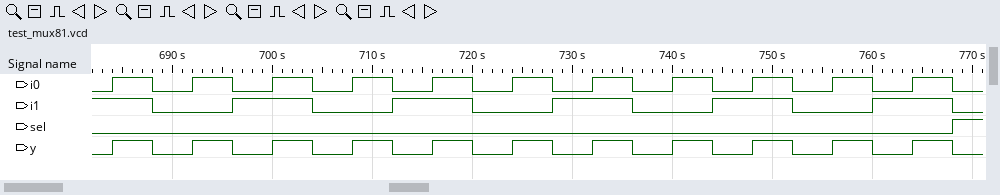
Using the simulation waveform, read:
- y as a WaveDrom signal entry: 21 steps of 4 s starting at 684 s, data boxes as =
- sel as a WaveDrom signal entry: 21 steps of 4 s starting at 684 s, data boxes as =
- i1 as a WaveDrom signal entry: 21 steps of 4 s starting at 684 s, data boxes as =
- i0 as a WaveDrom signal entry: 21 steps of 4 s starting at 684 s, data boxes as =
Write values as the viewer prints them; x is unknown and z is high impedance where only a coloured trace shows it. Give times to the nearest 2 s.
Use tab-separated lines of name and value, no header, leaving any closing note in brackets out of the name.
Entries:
y as a WaveDrom signal entry: 21 steps of 4 s starting at 684 s, data boxes as =	{name: 'y', wave: '101010101010101010101'}
sel as a WaveDrom signal entry: 21 steps of 4 s starting at 684 s, data boxes as =	{name: 'sel', wave: '0....................'}
i1 as a WaveDrom signal entry: 21 steps of 4 s starting at 684 s, data boxes as =	{name: 'i1', wave: '10.1.0.1.0.1.0.1.0.1.'}
i0 as a WaveDrom signal entry: 21 steps of 4 s starting at 684 s, data boxes as =	{name: 'i0', wave: '101010101010101010101'}
